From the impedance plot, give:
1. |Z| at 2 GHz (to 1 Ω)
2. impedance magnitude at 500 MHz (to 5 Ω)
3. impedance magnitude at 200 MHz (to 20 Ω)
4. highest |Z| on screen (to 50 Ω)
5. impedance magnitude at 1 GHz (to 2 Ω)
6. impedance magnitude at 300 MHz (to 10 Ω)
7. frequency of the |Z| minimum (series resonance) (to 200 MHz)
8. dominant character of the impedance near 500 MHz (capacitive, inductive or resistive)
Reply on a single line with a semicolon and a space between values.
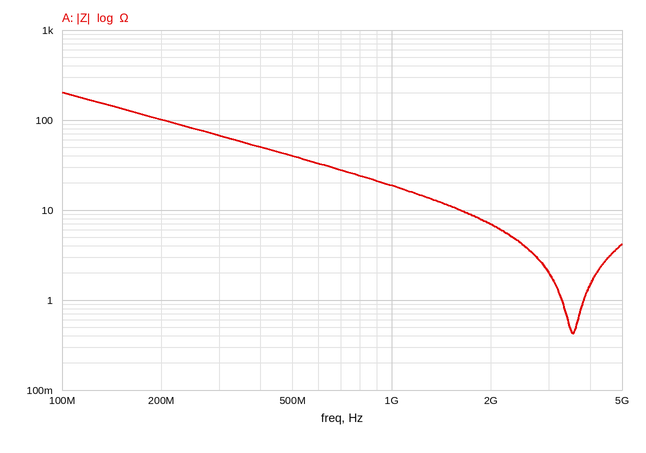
7 Ω; 40 Ω; 100 Ω; 200 Ω; 18 Ω; 70 Ω; 3.6 GHz; capacitive
